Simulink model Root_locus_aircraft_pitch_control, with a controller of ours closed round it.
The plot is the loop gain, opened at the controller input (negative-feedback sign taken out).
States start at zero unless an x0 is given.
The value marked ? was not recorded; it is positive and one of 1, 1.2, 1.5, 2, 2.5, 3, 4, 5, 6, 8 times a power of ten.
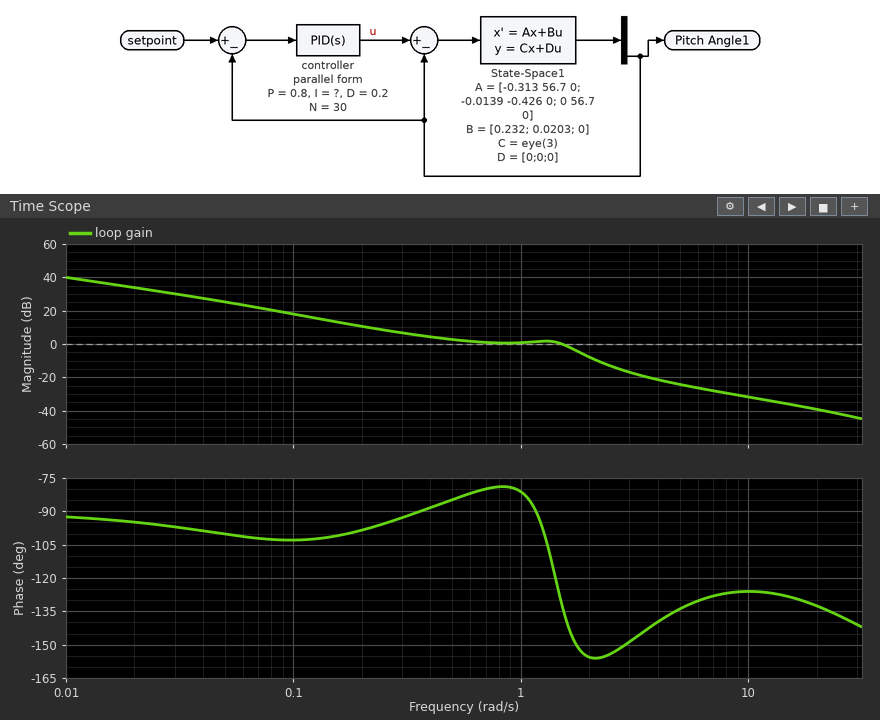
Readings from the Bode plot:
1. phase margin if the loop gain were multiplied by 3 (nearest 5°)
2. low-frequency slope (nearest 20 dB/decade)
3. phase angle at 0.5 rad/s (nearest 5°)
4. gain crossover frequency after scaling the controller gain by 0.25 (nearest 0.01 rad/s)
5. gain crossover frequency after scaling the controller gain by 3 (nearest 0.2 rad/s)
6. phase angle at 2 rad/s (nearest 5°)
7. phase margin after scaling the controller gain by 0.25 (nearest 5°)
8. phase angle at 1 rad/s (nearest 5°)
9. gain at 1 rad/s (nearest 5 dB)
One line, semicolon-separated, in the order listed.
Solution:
25°; -20 dB/decade; -85°; 0.17 rad/s; 2.2 rad/s; -155°; 80°; -80°; 0 dB
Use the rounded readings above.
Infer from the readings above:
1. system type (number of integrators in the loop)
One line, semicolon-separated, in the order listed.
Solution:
1
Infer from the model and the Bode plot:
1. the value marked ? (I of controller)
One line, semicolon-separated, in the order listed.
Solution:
1
